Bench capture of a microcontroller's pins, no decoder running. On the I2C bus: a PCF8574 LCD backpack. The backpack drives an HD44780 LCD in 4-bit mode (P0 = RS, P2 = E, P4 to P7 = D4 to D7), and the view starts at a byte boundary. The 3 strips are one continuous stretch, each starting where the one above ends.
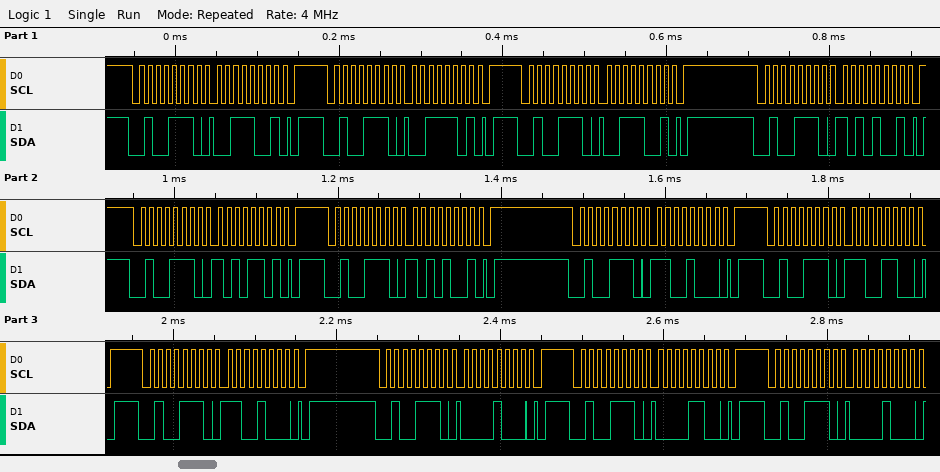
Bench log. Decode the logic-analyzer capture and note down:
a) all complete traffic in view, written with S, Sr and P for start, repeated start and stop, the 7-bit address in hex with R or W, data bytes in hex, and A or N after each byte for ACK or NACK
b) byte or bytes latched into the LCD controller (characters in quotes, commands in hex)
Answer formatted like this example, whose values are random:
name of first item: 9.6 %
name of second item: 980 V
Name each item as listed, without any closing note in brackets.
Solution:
all complete traffic in view, written with S, Sr and P for start, repeated start and stop, the 7-bit address in hex with R or W, data bytes in hex, and A or N after each byte for ACK or NACK: S 27W A 39 A P S 27W A 3D A P S 27W A 39 A P S 27W A A9 A P S 27W A AD A P S 27W A A9 A P S 27W A C8 A P S 27W A CC A P S 27W A C8 A P S 27W A 08 A P S 27W A 0C A P S 27W A 08 A
byte or bytes latched into the LCD controller: ':' 0xC0
